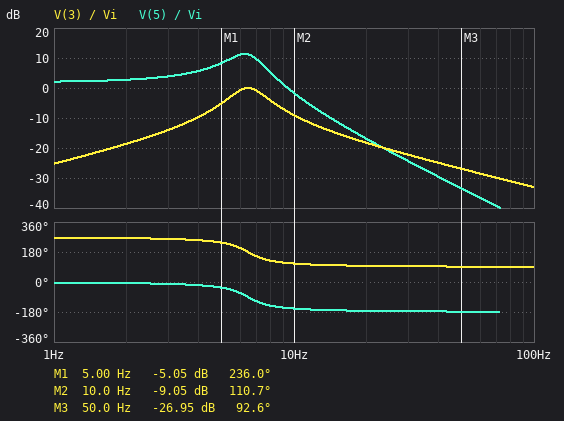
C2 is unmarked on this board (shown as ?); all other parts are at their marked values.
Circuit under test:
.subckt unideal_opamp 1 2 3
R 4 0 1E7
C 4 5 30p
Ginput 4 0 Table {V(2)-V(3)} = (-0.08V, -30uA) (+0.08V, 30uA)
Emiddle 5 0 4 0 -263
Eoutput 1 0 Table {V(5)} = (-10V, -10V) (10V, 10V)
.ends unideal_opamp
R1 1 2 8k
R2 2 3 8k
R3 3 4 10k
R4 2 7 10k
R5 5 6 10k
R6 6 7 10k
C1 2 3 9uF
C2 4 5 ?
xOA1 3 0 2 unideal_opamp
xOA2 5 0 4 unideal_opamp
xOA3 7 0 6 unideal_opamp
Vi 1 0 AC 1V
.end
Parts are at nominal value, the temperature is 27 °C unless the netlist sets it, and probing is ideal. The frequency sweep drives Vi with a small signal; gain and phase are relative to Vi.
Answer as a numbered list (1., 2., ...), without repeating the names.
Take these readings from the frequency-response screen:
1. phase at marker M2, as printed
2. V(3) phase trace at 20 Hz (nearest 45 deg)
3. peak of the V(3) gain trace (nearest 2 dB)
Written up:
1. 110.7 deg
2. 90 deg
3. 0 dB
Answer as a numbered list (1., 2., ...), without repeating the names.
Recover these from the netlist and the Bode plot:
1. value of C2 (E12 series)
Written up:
1. 680 nF
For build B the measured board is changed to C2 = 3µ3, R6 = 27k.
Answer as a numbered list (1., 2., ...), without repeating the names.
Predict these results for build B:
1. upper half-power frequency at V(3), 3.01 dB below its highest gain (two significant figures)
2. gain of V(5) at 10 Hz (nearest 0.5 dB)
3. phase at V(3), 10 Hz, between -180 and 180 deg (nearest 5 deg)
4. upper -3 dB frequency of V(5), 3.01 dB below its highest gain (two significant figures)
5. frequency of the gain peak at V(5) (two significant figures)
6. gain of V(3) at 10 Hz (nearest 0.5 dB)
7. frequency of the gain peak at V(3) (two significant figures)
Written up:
1. 6.0 Hz
2. -17.5 dB
3. 105 deg
4. 5.6 Hz
5. 4.5 Hz
6. -11.0 dB
7. 4.8 Hz
